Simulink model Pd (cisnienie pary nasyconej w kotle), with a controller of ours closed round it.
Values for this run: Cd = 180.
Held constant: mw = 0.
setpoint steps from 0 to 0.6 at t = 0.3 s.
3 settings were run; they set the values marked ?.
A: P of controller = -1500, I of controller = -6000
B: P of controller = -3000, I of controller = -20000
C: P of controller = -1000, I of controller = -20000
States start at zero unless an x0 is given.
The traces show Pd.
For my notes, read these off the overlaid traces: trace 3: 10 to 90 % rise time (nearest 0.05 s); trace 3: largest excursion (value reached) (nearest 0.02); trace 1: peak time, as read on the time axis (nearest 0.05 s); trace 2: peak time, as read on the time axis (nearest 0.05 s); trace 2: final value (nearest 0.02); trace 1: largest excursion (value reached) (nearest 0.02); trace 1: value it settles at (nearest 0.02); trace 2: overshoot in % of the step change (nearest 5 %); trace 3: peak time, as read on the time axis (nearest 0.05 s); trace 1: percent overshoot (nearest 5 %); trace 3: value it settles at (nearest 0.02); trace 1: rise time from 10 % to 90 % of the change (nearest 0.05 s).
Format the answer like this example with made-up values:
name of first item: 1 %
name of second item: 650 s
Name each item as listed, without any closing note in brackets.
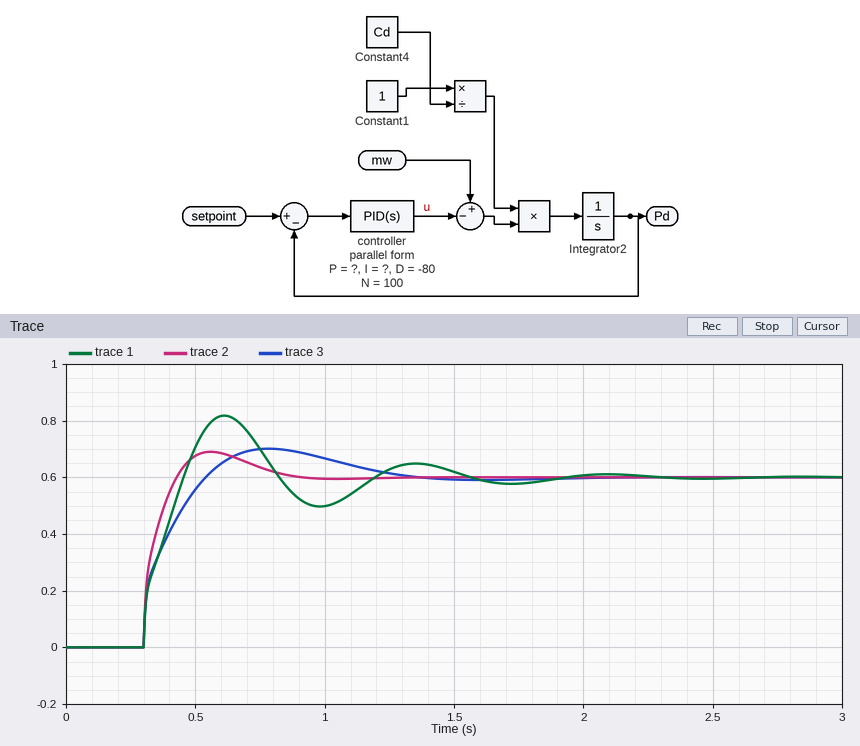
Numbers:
trace 3: 10 to 90 % rise time: 0.20 s
trace 3: largest excursion (value reached): 0.70
trace 1: peak time, as read on the time axis: 0.60 s
trace 2: peak time, as read on the time axis: 0.55 s
trace 2: final value: 0.60
trace 1: largest excursion (value reached): 0.82
trace 1: value it settles at: 0.60
trace 2: overshoot in % of the step change: 15 %
trace 3: peak time, as read on the time axis: 0.80 s
trace 1: percent overshoot: 35 %
trace 3: value it settles at: 0.60
trace 1: rise time from 10 % to 90 % of the change: 0.15 s
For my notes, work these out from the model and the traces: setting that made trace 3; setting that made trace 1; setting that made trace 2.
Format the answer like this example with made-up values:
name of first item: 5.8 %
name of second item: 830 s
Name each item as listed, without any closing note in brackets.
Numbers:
setting that made trace 3: A
setting that made trace 1: C
setting that made trace 2: B
